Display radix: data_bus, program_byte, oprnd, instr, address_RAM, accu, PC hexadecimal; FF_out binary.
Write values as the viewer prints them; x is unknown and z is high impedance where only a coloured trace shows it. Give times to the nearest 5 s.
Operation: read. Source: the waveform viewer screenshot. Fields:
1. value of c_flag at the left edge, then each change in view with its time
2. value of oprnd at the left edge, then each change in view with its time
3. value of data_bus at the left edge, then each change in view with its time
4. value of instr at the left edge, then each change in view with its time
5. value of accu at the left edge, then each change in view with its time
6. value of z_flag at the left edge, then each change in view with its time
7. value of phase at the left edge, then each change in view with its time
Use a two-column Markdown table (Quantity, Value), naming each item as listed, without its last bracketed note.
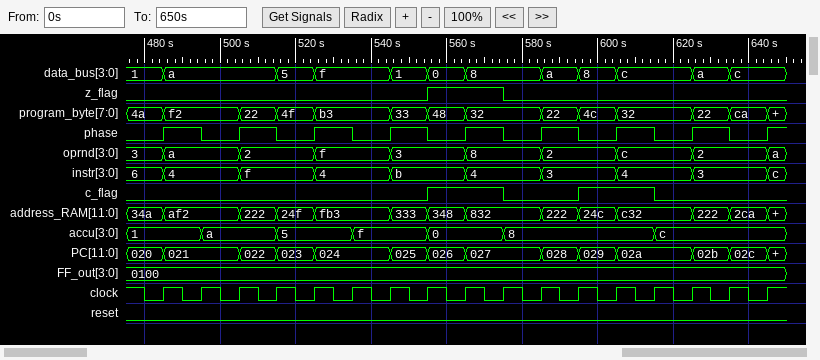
| Quantity | Value |
|---|---|
| value of c_flag at the left edge, then each change in view with its time | 0, 1 at 555 s, 0 at 575 s, 1 at 595 s, 0 at 615 s |
| value of oprnd at the left edge, then each change in view with its time | 3, a at 485 s, 2 at 505 s, f at 525 s, 3 at 545 s, 8 at 565 s, 2 at 585 s, c at 605 s, 2 at 625 s, a at 645 s |
| value of data_bus at the left edge, then each change in view with its time | 1, a at 485 s, 5 at 515 s, f at 525 s, 1 at 545 s, 0 at 555 s, 8 at 565 s, a at 585 s, 8 at 595 s, c at 605 s, a at 625 s, c at 635 s |
| value of instr at the left edge, then each change in view with its time | 6, 4 at 485 s, f at 505 s, 4 at 525 s, b at 545 s, 4 at 565 s, 3 at 585 s, 4 at 605 s, 3 at 625 s, c at 645 s |
| value of accu at the left edge, then each change in view with its time | 1, a at 495 s, 5 at 515 s, f at 535 s, 0 at 555 s, 8 at 575 s, c at 615 s |
| value of z_flag at the left edge, then each change in view with its time | 0, 1 at 555 s, 0 at 575 s |
| value of phase at the left edge, then each change in view with its time | 0, 1 at 485 s, 0 at 495 s, 1 at 505 s, 0 at 515 s, 1 at 525 s, 0 at 535 s, 1 at 545 s, 0 at 555 s, 1 at 565 s, 0 at 575 s, 1 at 585 s, 0 at 595 s, 1 at 605 s, 0 at 615 s, 1 at 625 s, 0 at 635 s, 1 at 645 s |
